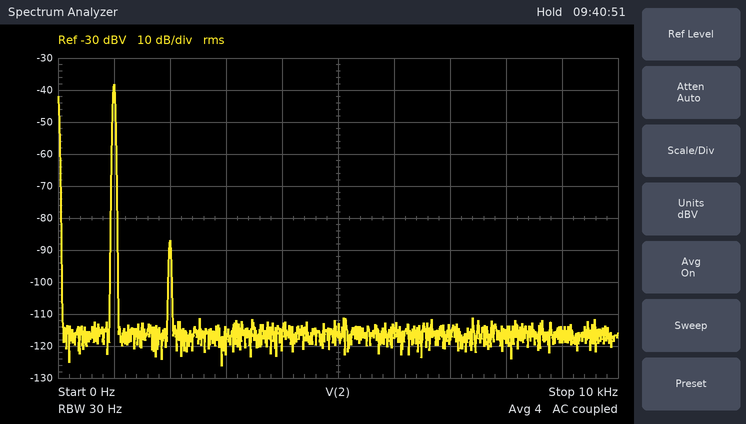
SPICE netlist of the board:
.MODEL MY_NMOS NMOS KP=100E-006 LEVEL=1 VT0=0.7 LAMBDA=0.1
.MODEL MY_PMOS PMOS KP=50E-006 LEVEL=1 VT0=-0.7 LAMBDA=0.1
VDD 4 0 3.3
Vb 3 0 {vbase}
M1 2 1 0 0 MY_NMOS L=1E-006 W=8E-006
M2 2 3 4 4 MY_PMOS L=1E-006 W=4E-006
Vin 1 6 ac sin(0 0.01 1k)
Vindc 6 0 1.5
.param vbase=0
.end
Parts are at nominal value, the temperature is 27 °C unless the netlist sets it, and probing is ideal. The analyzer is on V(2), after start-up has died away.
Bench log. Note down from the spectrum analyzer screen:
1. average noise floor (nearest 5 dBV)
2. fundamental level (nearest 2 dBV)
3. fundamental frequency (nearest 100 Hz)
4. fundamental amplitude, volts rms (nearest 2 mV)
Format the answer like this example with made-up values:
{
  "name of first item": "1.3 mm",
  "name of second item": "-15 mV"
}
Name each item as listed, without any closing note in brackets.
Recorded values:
{
  "average noise floor": "-115 dBV",
  "fundamental level": "-38 dBV",
  "fundamental frequency": "1.0 kHz",
  "fundamental amplitude, volts rms": "12 mV"
}
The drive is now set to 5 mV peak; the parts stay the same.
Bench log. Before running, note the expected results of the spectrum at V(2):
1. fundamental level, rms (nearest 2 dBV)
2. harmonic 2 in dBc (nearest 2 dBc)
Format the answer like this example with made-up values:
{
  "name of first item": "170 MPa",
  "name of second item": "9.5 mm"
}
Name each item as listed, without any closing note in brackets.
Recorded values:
{
  "fundamental level, rms": "-44 dBV",
  "harmonic 2 in dBc": "-54 dBc"
}
